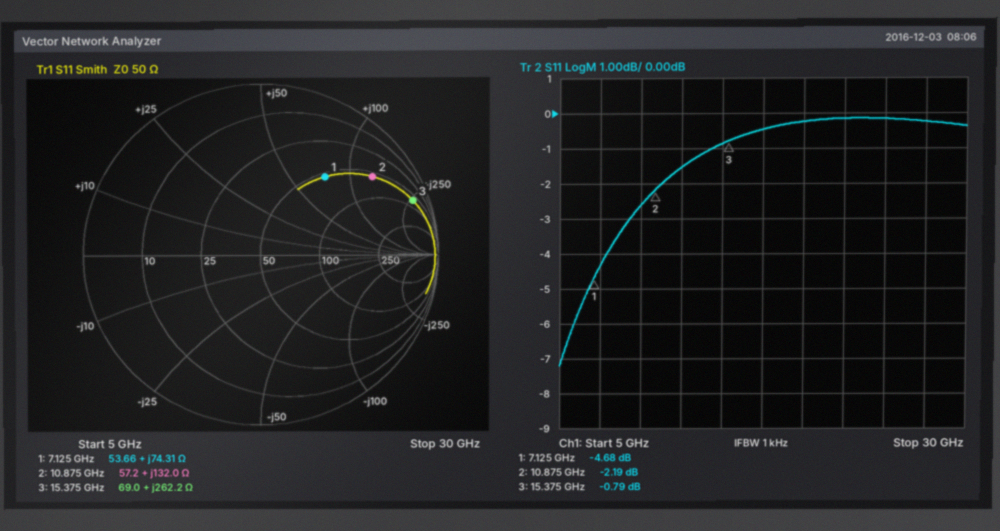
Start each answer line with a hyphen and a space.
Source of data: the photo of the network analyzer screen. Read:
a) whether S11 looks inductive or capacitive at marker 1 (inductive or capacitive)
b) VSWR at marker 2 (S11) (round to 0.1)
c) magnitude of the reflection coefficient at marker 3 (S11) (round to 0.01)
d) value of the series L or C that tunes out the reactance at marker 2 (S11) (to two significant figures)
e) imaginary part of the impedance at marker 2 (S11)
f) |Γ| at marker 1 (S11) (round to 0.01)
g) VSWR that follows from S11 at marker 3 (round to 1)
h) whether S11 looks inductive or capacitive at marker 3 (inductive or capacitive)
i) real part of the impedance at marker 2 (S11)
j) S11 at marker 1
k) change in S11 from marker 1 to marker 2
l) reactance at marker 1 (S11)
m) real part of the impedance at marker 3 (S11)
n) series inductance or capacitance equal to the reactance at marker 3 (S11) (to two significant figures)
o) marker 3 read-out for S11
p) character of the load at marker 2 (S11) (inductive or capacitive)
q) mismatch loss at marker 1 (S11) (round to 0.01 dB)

- inductive
- 8.0
- 0.91
- 110 fF
- +132.0 Ω
- 0.58
- 22
- inductive
- 57.2 Ω
- -4.68 dB
- 2.49 dB
- +74.31 Ω
- 69.0 Ω
- 2.7 nH
- -0.79 dB
- inductive
- 1.81 dB
